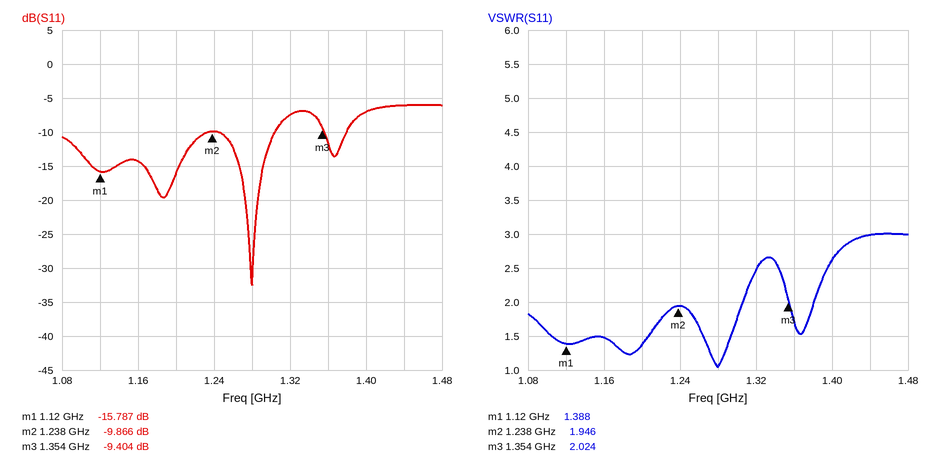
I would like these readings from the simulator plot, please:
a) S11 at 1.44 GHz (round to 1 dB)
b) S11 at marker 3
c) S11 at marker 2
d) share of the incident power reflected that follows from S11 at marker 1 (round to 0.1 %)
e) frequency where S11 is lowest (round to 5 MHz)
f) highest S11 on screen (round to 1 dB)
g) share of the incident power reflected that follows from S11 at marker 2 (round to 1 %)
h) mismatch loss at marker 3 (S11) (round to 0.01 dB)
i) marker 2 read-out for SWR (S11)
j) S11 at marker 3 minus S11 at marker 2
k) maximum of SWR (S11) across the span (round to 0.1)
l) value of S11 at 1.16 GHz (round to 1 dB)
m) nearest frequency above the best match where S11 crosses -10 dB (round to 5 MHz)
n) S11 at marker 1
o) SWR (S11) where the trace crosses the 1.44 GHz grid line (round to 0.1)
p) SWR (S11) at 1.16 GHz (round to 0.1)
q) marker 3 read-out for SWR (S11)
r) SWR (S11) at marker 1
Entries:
-6 dB
-9.404 dB
-9.866 dB
2.6 %
1.280 GHz
-6 dB
10 %
0.53 dB
1.946
0.462 dB
3.0
-14 dB
1.305 GHz
-15.787 dB
3.0
1.5
2.024
1.388
